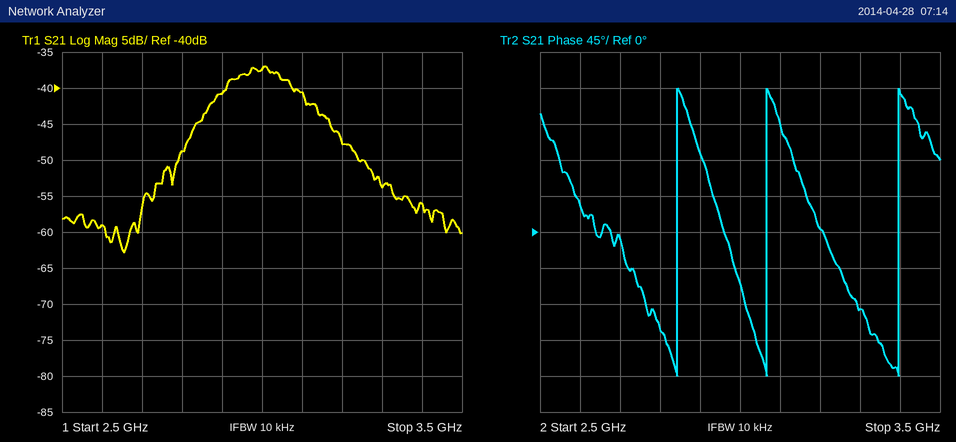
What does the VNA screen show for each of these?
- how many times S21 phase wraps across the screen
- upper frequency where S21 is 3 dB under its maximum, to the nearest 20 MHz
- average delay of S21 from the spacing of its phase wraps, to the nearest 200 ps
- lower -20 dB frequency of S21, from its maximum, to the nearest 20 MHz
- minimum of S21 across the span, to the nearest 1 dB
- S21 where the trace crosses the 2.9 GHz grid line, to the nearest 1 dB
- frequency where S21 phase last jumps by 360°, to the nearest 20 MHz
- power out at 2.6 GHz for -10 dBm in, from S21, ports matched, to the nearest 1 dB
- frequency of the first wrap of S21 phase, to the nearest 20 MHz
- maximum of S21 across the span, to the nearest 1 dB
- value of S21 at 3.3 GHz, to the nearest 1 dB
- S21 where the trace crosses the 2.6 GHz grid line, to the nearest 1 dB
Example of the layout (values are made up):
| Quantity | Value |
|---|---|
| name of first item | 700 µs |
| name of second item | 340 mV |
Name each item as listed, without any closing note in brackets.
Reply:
| Quantity | Value |
|---|---|
| how many times S21 phase wraps across the screen | 3 |
| upper frequency where S21 is 3 dB under its maximum, to the nearest 20 MHz | 3.08 GHz |
| average delay of S21 from the spacing of its phase wraps, to the nearest 200 ps | 3.6 ns |
| lower -20 dB frequency of S21, from its maximum, to the nearest 20 MHz | 2.70 GHz |
| minimum of S21 across the span, to the nearest 1 dB | -63 dB |
| S21 where the trace crosses the 2.9 GHz grid line, to the nearest 1 dB | -41 dB |
| frequency where S21 phase last jumps by 360°, to the nearest 20 MHz | 3.40 GHz |
| power out at 2.6 GHz for -10 dBm in, from S21, ports matched, to the nearest 1 dB | -69 dBm |
| frequency of the first wrap of S21 phase, to the nearest 20 MHz | 2.84 GHz |
| maximum of S21 across the span, to the nearest 1 dB | -37 dB |
| value of S21 at 3.3 GHz, to the nearest 1 dB | -54 dB |
| S21 where the trace crosses the 2.6 GHz grid line, to the nearest 1 dB | -59 dB |
